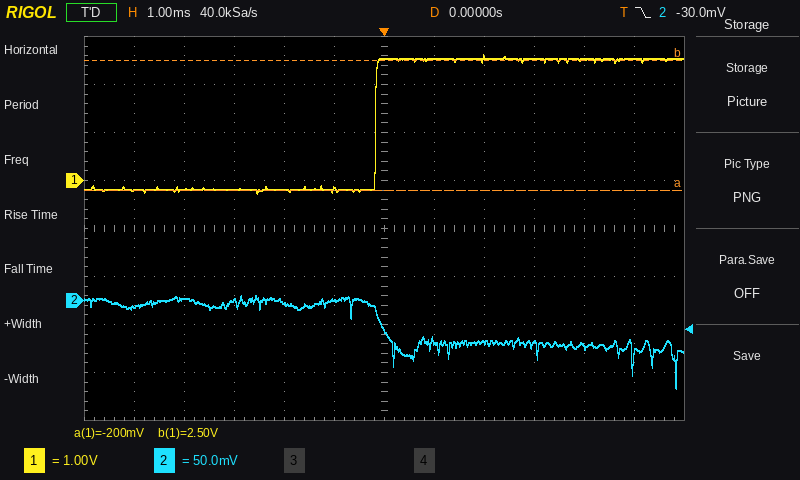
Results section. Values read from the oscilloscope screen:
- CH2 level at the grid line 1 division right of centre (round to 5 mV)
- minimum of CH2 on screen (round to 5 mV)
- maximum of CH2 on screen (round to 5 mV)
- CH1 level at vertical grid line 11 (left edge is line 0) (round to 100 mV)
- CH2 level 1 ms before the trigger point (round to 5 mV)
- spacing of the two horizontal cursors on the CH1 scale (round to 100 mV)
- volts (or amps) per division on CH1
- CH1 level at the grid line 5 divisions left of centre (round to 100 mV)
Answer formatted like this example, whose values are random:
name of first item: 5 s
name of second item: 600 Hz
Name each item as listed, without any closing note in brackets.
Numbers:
CH2 level at the grid line 1 division right of centre: -40 mV
minimum of CH2 on screen: -90 mV
maximum of CH2 on screen: 5 mV
CH1 level at vertical grid line 11 (left edge is line 0): 2.5 V
CH2 level 1 ms before the trigger point: 0 mV
spacing of the two horizontal cursors on the CH1 scale: 2.7 V
volts (or amps) per division on CH1: 1 V
CH1 level at the grid line 5 divisions left of centre: -200 mV
